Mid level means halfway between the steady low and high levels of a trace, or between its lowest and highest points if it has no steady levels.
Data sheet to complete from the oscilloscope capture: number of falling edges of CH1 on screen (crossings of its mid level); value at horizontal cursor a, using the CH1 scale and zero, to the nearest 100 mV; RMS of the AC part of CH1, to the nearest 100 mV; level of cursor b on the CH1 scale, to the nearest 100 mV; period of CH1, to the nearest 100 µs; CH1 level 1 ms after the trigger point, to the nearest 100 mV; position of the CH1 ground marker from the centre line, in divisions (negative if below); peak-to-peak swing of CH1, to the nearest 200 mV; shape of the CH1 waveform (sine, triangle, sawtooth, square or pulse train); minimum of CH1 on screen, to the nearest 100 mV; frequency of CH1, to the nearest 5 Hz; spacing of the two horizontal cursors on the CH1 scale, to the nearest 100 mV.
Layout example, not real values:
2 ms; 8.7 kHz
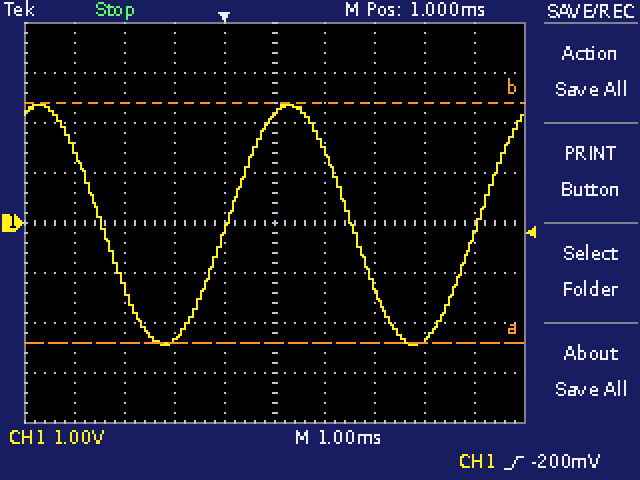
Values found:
2; -2.4 V; 1.7 V; 2.4 V; 5.0 ms; 2.2 V; 0.0 div; 4.8 V; sine; -2.4 V; 200 Hz; 4.8 V
